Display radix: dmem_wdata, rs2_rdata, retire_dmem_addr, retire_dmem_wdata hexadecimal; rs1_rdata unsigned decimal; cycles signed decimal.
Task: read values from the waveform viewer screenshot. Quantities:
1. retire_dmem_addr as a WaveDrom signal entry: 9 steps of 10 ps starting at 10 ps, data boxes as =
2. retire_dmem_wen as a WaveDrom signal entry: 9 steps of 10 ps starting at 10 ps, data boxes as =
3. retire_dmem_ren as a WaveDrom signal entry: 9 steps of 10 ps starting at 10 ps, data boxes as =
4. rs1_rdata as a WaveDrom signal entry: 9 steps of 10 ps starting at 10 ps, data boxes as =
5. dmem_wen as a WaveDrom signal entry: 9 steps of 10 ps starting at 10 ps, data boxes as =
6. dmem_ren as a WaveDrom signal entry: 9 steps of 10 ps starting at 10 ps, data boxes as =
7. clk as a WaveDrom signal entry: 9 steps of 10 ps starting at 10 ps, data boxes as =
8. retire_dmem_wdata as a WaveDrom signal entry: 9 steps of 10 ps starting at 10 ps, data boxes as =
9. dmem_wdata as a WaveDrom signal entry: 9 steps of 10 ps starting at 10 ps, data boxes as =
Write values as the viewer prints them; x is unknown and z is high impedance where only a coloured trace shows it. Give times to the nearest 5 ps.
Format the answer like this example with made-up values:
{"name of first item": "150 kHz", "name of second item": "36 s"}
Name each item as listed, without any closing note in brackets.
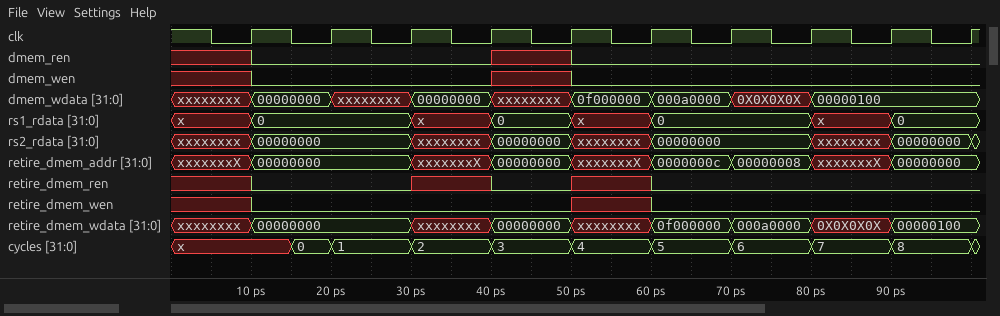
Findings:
{"retire_dmem_addr as a WaveDrom signal entry: 9 steps of 10 ps starting at 10 ps, data boxes as =": "{name: 'retire_dmem_addr', wave: '=.=======', data: '00000000 xxxxxxxX 00000000 xxxxxxxX 0000000c 00000008 xxxxxxxX 00000000'}", "retire_dmem_wen as a WaveDrom signal entry: 9 steps of 10 ps starting at 10 ps, data boxes as =": "{name: 'retire_dmem_wen', wave: '0...x0...'}", "retire_dmem_ren as a WaveDrom signal entry: 9 steps of 10 ps starting at 10 ps, data boxes as =": "{name: 'retire_dmem_ren', wave: '0.x0x0...'}", "rs1_rdata as a WaveDrom signal entry: 9 steps of 10 ps starting at 10 ps, data boxes as =": "{name: 'rs1_rdata', wave: '=.x=x=.x=', data: '0 0 0 0'}", "dmem_wen as a WaveDrom signal entry: 9 steps of 10 ps starting at 10 ps, data boxes as =": "{name: 'dmem_wen', wave: '0..x0....'}", "dmem_ren as a WaveDrom signal entry: 9 steps of 10 ps starting at 10 ps, data boxes as =": "{name: 'dmem_ren', wave: '0..x0....'}", "clk as a WaveDrom signal entry: 9 steps of 10 ps starting at 10 ps, data boxes as =": "{name: 'clk', wave: 'p........'}", "retire_dmem_wdata as a WaveDrom signal entry: 9 steps of 10 ps starting at 10 ps, data boxes as =": "{name: 'retire_dmem_wdata', wave: '=.x=x====', data: '00000000 00000000 0f000000 000a0000 0X0X0X0X 00000100'}", "dmem_wdata as a WaveDrom signal entry: 9 steps of 10 ps starting at 10 ps, data boxes as =": "{name: 'dmem_wdata', wave: '=x=x====.', data: '00000000 00000000 0f000000 000a0000 0X0X0X0X 00000100'}"}
